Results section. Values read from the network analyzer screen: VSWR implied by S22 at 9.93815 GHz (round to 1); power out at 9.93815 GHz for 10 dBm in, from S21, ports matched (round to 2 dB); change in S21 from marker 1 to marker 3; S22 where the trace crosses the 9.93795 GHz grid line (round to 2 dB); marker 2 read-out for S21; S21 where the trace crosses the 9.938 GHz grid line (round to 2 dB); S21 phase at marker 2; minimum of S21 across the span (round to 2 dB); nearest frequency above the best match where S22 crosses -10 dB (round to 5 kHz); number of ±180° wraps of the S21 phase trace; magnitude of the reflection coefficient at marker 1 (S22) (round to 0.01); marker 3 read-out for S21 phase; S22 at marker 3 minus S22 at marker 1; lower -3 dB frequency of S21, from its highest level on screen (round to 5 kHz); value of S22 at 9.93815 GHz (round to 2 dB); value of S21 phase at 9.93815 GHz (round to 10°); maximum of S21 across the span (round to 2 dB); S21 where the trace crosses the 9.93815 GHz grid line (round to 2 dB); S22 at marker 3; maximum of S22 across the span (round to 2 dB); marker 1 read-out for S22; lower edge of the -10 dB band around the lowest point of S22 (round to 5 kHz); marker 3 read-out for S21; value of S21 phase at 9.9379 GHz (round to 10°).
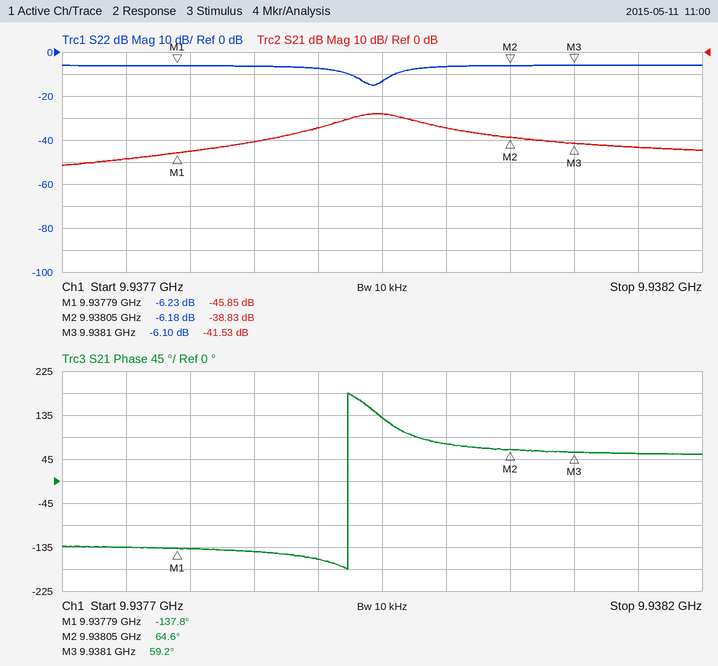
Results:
3
-34 dBm
4.32 dB
-14 dB
-38.83 dB
-34 dB
64.6°
-52 dB
9.937960 GHz
1
0.49
59.2°
0.13 dB
9.937920 GHz
-6 dB
60°
-28 dB
-44 dB
-6.10 dB
-6 dB
-6.23 dB
9.937925 GHz
-41.53 dB
-160°
